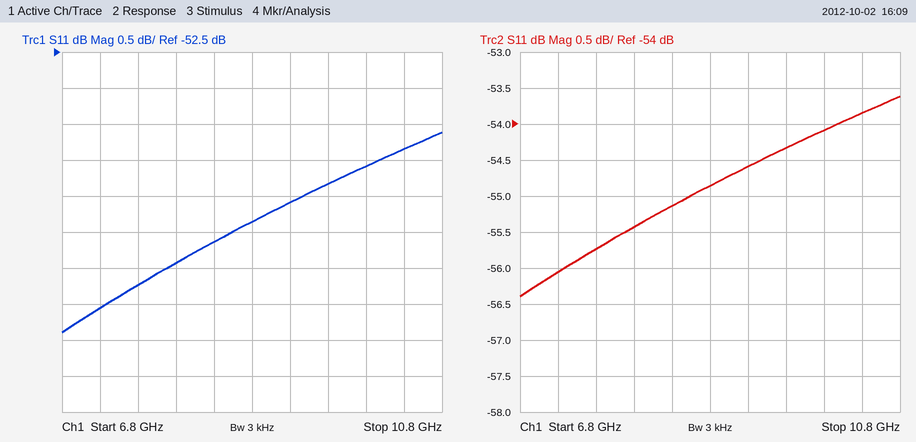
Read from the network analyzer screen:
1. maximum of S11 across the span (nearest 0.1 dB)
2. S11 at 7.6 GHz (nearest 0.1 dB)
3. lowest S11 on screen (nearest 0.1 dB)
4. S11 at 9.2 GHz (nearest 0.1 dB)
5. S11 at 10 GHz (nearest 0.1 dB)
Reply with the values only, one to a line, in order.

-53.6 dB
-55.7 dB
-56.4 dB
-54.6 dB
-54.1 dB
